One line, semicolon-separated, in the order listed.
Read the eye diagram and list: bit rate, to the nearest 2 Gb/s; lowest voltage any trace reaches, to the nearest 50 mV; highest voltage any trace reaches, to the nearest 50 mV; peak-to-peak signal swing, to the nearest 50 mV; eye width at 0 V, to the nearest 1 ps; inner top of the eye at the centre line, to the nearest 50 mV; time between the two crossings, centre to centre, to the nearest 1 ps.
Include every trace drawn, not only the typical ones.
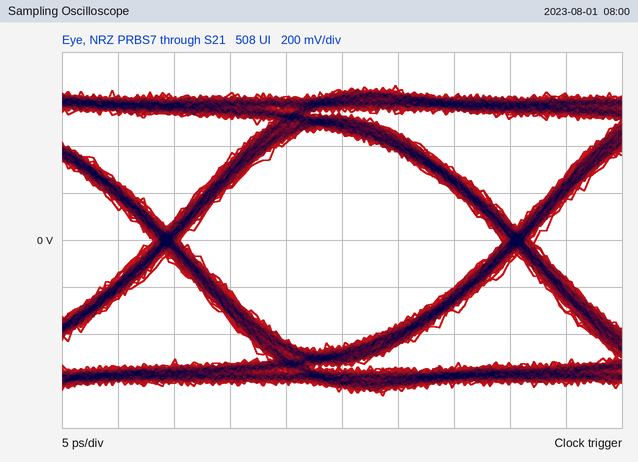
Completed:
32 Gb/s; -650 mV; 650 mV; 1.30 V; 29 ps; 450 mV; 31 ps
